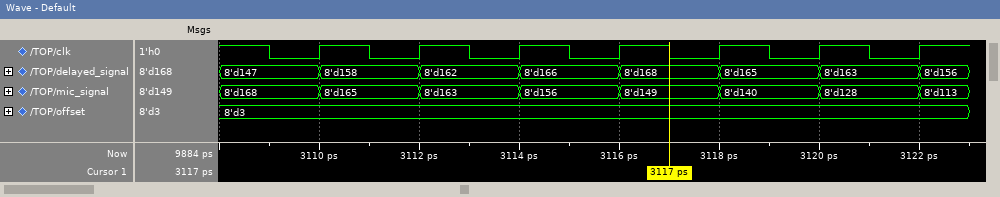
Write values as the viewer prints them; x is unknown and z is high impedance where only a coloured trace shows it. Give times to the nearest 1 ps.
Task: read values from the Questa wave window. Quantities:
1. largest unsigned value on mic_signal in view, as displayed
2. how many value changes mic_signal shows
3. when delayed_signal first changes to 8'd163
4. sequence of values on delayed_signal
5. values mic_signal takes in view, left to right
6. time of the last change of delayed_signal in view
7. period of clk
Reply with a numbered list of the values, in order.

1. 8'd168
2. 7
3. 3120 ps
4. 8'd147, 8'd158, 8'd162, 8'd166, 8'd168, 8'd165, 8'd163, 8'd156
5. 8'd168, 8'd165, 8'd163, 8'd156, 8'd149, 8'd140, 8'd128, 8'd113
6. 3122 ps
7. 2 ps
